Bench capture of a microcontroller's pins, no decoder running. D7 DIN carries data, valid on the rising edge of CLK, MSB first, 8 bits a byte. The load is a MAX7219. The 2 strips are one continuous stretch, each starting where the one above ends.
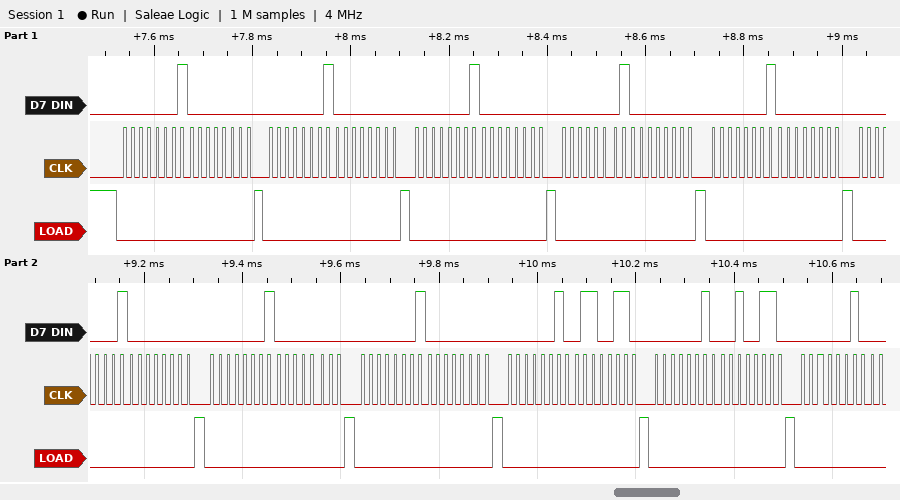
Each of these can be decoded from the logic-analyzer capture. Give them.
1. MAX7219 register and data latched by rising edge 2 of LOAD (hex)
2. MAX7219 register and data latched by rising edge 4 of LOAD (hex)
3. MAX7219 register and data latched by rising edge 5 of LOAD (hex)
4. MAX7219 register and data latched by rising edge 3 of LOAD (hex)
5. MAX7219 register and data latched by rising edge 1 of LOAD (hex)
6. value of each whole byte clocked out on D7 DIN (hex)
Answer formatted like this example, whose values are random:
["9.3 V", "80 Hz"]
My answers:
["register 0x1, data 0x00", "register 0x1, data 0x00", "register 0x1, data 0x00", "register 0x1, data 0x00", "register 0x1, data 0x00", "01 00 01 00 01 00 01 00 01 00 01 00 01 00 01 00 02 66 02 26 02"]
